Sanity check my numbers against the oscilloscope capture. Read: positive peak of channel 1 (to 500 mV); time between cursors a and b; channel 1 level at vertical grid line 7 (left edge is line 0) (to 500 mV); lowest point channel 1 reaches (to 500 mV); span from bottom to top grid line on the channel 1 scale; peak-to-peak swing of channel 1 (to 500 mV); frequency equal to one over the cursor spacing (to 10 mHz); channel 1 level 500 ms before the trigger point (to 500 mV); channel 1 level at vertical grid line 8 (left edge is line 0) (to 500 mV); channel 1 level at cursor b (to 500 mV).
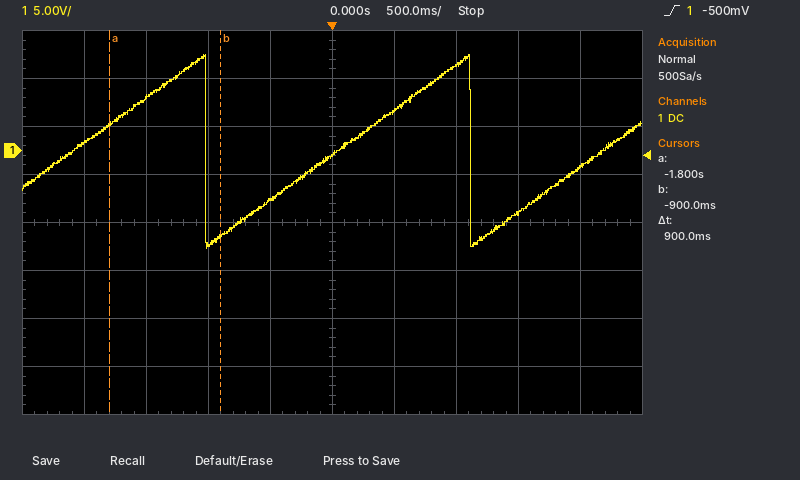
10.0 V
900 ms
9.0 V
-10.0 V
40 V
20.0 V
1.11 Hz
-5.0 V
-6.5 V
-9.0 V
